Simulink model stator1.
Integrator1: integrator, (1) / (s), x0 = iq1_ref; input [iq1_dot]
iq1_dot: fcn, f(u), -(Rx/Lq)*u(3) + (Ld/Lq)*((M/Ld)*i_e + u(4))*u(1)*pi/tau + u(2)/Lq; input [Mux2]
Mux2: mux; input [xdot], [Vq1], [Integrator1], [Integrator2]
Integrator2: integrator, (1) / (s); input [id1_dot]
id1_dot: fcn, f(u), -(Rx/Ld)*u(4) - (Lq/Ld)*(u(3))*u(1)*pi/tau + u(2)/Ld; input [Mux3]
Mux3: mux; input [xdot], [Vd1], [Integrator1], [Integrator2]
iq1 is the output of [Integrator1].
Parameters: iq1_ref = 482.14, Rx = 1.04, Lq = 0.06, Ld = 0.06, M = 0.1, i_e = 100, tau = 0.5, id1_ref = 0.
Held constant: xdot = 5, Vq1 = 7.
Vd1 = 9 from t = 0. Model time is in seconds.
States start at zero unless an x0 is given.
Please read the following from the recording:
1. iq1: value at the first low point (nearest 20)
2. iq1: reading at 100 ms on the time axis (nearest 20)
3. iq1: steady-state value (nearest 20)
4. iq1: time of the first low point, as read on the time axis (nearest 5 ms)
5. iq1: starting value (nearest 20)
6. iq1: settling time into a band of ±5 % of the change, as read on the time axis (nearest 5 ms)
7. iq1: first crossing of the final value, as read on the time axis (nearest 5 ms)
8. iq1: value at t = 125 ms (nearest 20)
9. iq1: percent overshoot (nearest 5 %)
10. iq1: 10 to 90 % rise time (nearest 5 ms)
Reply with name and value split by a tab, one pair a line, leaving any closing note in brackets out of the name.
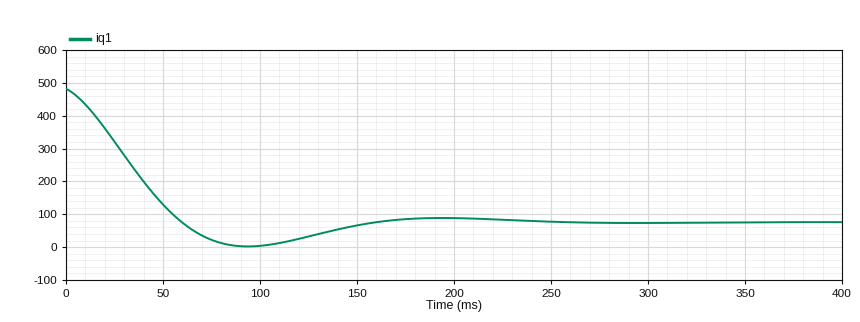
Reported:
iq1: value at the first low point	0
iq1: reading at 100 ms on the time axis	0
iq1: steady-state value	80
iq1: time of the first low point, as read on the time axis	95 ms
iq1: starting value	480
iq1: settling time into a band of ±5 % of the change, as read on the time axis	140 ms
iq1: first crossing of the final value, as read on the time axis	60 ms
iq1: value at t = 125 ms	40
iq1: percent overshoot	20 %
iq1: 10 to 90 % rise time	45 ms
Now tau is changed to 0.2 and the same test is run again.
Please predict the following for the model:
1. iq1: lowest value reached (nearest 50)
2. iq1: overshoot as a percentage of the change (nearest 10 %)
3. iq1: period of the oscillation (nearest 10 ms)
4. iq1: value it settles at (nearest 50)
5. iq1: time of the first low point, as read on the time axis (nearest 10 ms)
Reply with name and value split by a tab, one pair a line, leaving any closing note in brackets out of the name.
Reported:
iq1: lowest value reached	-200
iq1: overshoot as a percentage of the change	50 %
iq1: period of the oscillation	80 ms
iq1: value it settles at	50
iq1: time of the first low point, as read on the time axis	40 ms
